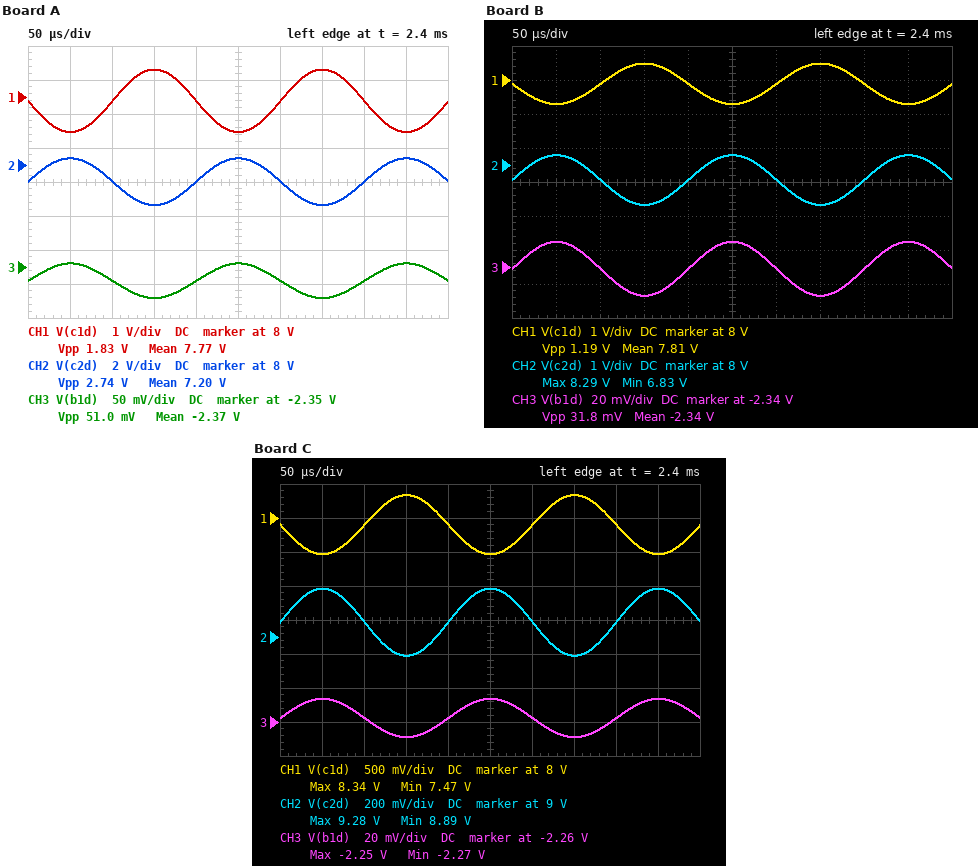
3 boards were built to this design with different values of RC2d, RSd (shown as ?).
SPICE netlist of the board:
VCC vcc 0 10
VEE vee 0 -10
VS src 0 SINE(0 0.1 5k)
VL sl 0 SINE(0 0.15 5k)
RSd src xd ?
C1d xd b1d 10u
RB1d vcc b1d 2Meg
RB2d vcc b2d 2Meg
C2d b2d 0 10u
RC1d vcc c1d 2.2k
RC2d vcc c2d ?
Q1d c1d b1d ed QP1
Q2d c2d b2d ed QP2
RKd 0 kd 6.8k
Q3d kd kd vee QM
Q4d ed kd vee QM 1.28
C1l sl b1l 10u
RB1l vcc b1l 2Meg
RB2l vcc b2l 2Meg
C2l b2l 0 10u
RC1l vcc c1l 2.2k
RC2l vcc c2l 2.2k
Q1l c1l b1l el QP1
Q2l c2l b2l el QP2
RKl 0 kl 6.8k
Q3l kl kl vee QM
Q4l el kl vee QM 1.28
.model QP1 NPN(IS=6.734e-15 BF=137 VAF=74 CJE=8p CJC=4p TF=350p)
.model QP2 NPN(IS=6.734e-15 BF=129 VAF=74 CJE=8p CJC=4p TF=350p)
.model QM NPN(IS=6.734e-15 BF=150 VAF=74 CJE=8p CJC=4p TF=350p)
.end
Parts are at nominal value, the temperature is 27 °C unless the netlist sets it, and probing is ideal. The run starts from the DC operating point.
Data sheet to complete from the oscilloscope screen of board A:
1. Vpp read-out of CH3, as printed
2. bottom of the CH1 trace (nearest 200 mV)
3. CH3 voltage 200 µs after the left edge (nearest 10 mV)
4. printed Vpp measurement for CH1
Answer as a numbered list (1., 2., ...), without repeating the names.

1. 51.0 mV
2. 7.0 V
3. -2.37 V
4. 1.83 V
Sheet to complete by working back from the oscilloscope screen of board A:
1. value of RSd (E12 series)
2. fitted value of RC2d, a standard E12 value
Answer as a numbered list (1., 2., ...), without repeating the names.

1. 27 kΩ
2. 3.3 kΩ
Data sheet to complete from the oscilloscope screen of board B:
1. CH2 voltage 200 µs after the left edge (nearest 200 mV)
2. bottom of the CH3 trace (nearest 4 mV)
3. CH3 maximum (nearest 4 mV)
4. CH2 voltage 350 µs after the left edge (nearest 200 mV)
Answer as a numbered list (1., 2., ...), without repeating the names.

1. 7.6 V
2. -2.356 V
3. -2.324 V
4. 6.8 V
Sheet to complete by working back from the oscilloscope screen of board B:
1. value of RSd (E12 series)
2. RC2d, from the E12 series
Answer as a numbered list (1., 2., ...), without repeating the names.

1. 47 kΩ
2. 2.7 kΩ
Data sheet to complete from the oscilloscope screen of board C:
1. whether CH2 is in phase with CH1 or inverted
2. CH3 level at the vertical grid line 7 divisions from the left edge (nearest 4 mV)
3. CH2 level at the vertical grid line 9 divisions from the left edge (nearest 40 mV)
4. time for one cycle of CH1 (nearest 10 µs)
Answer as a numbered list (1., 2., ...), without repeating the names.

1. inverted
2. -2.268 V
3. 9.28 V
4. 200 µs
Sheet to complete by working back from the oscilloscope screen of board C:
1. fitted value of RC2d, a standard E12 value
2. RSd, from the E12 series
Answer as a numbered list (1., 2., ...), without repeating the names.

1. 1 kΩ
2. 68 kΩ
